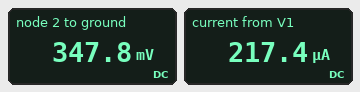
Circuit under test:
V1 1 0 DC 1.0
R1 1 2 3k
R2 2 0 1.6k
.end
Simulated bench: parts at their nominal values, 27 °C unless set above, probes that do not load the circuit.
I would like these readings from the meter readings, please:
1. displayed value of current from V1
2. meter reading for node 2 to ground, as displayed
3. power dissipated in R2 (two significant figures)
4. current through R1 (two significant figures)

217.4 µA
347.8 mV
76 µW
220 µA
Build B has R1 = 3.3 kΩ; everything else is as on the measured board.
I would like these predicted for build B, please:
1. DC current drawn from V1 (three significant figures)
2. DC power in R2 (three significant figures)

204 µA
66.6 µW
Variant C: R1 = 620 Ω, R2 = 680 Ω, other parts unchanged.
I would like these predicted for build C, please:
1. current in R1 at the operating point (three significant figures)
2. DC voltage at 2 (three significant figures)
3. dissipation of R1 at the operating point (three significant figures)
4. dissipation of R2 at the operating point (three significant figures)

769 µA
523 mV
367 µW
402 µW
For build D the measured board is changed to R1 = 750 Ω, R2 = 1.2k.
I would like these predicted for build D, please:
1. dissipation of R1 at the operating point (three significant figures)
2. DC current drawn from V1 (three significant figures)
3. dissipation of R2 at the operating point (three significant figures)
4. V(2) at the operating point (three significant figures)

197 µW
513 µA
316 µW
615 mV
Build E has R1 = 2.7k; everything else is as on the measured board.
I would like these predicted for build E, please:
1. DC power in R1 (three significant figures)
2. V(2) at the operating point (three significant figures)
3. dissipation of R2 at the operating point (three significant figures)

146 µW
372 mV
86.5 µW
